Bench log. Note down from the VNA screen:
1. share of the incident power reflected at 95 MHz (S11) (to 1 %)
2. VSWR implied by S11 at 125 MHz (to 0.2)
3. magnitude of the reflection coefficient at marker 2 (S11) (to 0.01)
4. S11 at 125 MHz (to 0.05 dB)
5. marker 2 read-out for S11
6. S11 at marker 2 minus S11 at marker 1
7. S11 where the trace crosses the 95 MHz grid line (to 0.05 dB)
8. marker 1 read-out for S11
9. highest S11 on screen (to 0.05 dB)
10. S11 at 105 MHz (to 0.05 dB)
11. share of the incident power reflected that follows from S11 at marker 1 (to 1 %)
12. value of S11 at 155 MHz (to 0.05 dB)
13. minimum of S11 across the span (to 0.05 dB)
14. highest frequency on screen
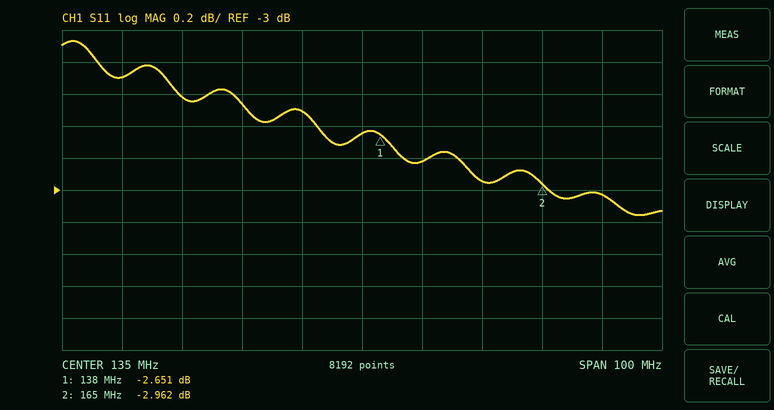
59 %
7.0
0.71
-2.50 dB
-2.962 dB
-0.311 dB
-2.30 dB
-2.651 dB
-2.05 dB
-2.40 dB
54 %
-2.95 dB
-3.15 dB
185 MHz
